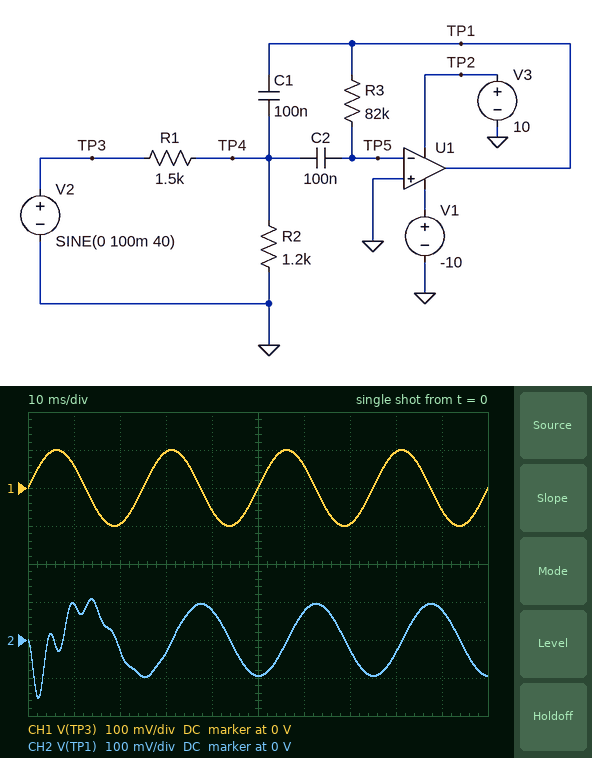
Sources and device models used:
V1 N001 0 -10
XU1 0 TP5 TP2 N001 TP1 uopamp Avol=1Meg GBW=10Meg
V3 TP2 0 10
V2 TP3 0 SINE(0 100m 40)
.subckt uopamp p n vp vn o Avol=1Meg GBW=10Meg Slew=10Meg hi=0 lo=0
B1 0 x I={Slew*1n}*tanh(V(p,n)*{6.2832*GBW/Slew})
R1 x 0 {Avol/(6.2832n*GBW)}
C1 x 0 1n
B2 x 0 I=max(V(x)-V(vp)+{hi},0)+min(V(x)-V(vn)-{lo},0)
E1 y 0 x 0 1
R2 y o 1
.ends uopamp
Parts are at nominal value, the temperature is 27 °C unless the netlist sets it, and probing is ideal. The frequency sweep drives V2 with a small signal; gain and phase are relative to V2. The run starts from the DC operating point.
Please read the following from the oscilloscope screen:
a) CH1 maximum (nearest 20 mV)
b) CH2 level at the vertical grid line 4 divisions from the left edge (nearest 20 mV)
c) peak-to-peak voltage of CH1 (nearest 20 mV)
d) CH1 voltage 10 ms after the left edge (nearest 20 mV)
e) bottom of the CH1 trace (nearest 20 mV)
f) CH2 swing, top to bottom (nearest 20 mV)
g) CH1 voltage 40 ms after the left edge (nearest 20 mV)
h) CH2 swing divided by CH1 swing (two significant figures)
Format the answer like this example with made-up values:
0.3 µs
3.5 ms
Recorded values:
100 mV
80 mV
200 mV
60 mV
-100 mV
260 mV
-60 mV
1.3
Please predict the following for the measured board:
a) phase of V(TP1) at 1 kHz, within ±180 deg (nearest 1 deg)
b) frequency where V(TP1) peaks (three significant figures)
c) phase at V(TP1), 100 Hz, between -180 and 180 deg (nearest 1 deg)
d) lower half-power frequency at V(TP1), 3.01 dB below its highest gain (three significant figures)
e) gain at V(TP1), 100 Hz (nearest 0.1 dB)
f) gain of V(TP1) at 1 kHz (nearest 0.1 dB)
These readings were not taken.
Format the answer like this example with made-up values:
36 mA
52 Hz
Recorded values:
92 deg
215 Hz
-96 deg
197 Hz
9.3 dB
0.9 dB
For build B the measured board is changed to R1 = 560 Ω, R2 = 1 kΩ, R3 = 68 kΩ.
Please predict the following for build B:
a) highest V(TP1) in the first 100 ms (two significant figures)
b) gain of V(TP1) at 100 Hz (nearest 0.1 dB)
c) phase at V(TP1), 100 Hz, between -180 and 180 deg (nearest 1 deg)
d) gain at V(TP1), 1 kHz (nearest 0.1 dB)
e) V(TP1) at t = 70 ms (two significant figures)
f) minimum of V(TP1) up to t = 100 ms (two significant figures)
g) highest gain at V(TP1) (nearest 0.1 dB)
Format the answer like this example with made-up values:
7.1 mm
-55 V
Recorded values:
130 mV
9.6 dB
-93 deg
10.0 dB
-32 mV
-190 mV
35.7 dB
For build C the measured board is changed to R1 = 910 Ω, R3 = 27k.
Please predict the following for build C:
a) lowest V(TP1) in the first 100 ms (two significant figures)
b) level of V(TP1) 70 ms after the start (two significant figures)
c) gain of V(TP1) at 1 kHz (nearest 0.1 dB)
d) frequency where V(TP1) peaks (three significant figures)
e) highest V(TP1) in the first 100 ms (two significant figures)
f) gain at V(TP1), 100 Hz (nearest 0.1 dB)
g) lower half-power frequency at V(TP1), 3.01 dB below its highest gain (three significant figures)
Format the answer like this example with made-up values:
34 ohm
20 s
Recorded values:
-63 mV
-11 mV
6.5 dB
426 Hz
39 mV
0.2 dB
371 Hz
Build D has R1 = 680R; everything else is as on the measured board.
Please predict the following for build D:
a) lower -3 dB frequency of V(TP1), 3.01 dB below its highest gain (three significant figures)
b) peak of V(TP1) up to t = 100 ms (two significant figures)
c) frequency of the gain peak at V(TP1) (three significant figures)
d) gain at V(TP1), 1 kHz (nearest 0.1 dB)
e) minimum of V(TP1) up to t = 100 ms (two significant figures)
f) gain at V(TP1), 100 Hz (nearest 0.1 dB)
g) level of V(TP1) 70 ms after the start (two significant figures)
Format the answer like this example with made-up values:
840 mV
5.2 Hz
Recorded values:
248 Hz
160 mV
267 Hz
8.0 dB
-230 mV
11.6 dB
-39 mV
